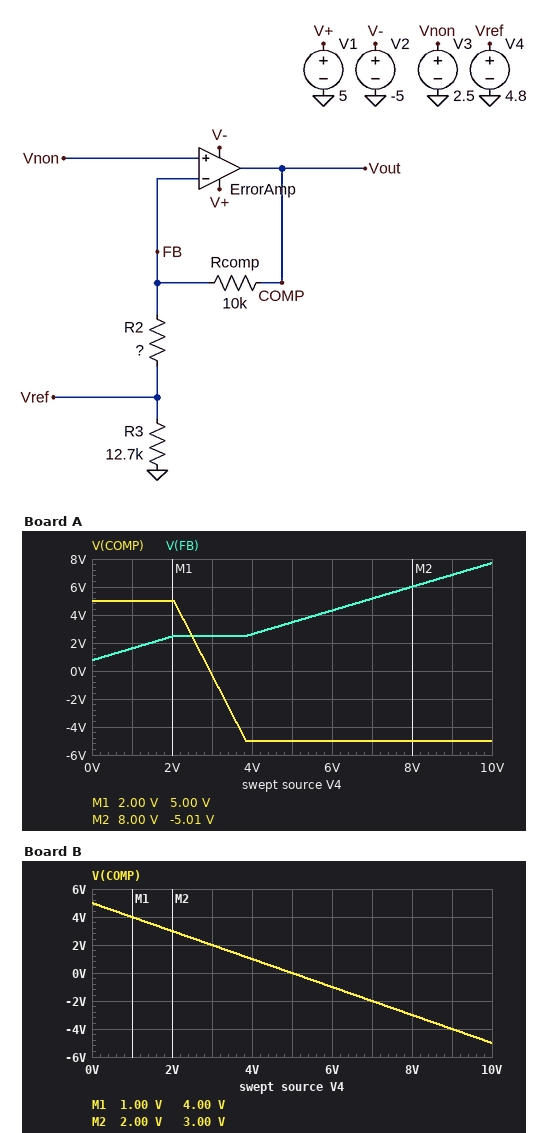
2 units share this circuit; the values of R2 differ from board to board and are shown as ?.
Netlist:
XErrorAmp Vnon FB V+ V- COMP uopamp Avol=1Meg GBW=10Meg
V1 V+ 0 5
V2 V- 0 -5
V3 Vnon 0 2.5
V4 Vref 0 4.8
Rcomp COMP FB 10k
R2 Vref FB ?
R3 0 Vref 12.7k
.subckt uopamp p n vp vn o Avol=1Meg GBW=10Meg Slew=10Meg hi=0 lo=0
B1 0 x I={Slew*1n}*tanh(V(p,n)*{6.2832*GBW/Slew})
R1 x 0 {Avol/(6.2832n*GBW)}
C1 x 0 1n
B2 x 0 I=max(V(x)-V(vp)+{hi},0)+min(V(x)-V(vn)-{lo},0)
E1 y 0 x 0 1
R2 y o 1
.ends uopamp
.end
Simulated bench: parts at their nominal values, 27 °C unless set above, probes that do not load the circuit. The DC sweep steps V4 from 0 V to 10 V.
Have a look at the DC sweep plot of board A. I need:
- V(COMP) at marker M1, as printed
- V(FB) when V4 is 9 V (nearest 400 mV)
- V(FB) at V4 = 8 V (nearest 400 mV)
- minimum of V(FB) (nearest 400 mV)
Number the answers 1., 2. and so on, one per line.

1. 5.00 V
2. 6.8 V
3. 6.0 V
4. 800 mV
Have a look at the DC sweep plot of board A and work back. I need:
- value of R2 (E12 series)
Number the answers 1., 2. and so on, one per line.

1. 1.8 kΩ
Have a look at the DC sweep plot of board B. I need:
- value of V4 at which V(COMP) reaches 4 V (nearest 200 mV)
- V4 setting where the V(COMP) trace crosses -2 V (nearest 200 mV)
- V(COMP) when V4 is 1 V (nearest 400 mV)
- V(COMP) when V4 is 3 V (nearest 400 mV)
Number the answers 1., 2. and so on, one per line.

1. 1.0 V
2. 7.0 V
3. 4.0 V
4. 2.0 V
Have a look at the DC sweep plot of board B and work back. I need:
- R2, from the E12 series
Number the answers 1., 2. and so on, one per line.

1. 10 kΩ
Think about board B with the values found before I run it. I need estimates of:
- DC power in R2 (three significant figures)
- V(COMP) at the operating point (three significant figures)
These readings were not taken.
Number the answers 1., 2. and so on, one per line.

1. 529 µW
2. 200 mV
